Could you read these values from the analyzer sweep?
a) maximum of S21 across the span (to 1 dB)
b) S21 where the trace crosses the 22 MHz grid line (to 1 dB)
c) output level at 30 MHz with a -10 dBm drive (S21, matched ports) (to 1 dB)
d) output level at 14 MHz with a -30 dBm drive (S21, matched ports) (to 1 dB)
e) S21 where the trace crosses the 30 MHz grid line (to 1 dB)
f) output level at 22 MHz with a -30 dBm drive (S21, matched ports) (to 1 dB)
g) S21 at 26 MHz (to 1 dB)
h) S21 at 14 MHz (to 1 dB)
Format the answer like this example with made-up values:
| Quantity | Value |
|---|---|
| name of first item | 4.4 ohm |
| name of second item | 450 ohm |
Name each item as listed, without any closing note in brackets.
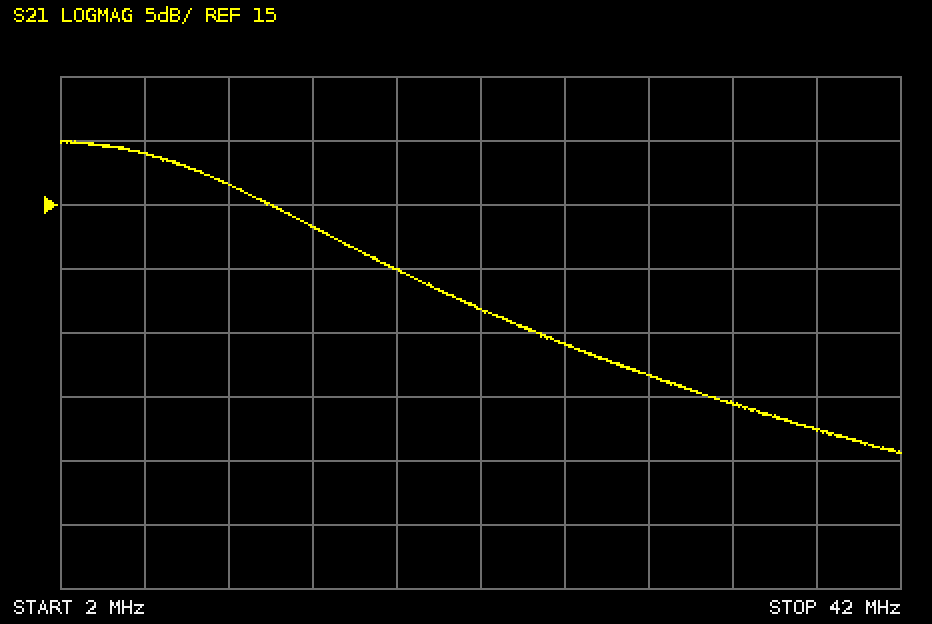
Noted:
| Quantity | Value |
|---|---|
| maximum of S21 across the span | 20 dB |
| S21 where the trace crosses the 22 MHz grid line | 7 dB |
| output level at 30 MHz with a -10 dBm drive (S21, matched ports) | -8 dBm |
| output level at 14 MHz with a -30 dBm drive (S21, matched ports) | -17 dBm |
| S21 where the trace crosses the 30 MHz grid line | 2 dB |
| output level at 22 MHz with a -30 dBm drive (S21, matched ports) | -23 dBm |
| S21 at 26 MHz | 4 dB |
| S21 at 14 MHz | 13 dB |
